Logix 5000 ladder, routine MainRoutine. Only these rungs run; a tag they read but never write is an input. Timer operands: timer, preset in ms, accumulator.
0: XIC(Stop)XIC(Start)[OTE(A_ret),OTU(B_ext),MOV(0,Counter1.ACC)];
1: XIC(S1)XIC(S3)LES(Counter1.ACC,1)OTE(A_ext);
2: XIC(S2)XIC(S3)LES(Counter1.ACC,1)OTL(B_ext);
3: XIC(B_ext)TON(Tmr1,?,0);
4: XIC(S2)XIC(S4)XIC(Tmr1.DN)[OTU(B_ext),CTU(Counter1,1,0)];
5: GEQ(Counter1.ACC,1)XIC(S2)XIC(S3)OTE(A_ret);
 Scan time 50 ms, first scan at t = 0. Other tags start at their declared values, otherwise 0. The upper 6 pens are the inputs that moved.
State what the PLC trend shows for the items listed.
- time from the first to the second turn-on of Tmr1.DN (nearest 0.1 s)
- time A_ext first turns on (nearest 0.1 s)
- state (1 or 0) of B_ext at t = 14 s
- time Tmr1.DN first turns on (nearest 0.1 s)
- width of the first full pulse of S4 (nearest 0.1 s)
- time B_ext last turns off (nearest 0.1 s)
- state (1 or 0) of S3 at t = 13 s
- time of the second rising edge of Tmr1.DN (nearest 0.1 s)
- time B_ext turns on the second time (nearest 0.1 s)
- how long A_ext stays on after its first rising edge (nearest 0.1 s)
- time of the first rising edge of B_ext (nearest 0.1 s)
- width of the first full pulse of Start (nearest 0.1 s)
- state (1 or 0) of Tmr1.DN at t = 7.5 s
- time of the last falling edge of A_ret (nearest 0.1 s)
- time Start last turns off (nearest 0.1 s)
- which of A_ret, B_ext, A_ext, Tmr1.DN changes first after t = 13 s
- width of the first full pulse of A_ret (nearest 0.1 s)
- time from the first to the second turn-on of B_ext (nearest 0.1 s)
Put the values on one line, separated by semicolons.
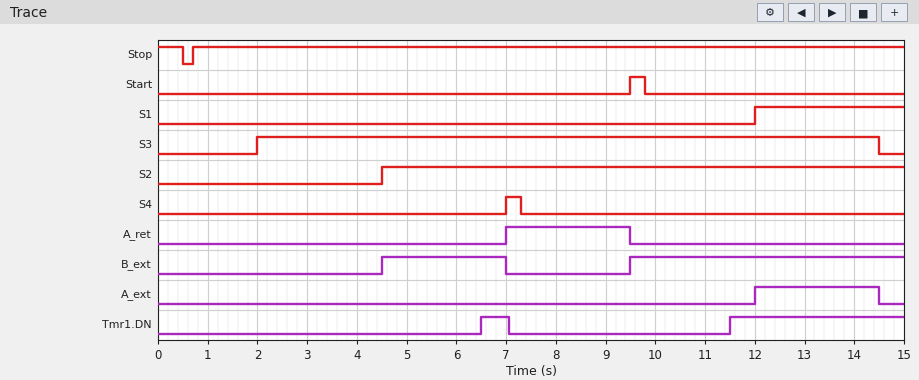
5.0 s; 12.0 s; 1; 6.5 s; 0.3 s; 7.0 s; 1; 11.5 s; 9.5 s; 2.5 s; 4.5 s; 0.3 s; 0; 9.5 s; 9.8 s; A_ext; 2.5 s; 5.0 s
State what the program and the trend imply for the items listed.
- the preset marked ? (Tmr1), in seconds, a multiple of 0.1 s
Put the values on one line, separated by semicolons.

2.0 s
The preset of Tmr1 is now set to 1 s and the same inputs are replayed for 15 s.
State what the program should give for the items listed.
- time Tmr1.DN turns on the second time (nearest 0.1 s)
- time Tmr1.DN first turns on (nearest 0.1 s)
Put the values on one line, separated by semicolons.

10.5 s; 5.5 s
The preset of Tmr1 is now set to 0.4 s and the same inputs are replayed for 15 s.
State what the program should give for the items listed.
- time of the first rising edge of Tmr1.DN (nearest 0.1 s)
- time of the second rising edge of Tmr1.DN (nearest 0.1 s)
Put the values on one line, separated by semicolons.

4.9 s; 9.9 s
